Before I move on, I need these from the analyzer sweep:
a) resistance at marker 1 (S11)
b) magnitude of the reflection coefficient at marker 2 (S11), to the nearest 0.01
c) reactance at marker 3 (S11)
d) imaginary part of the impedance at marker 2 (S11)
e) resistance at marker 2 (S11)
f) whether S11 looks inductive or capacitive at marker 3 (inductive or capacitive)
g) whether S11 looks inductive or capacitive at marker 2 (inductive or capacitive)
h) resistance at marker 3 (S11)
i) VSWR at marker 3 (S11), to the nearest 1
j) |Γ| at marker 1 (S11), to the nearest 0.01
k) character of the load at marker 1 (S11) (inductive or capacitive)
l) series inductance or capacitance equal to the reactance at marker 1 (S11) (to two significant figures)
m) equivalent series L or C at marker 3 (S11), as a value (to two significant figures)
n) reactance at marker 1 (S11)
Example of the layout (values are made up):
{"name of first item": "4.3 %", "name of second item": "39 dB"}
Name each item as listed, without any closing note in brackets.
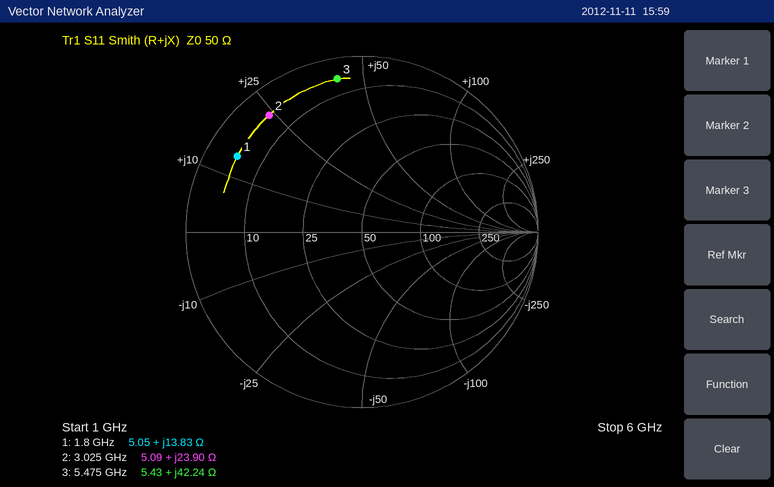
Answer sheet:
{"resistance at marker 1": "5.05 Ω", "magnitude of the reflection coefficient at marker 2 (S11), to the nearest 0.01": "0.85", "reactance at marker 3": "+42.24 Ω", "imaginary part of the impedance at marker 2": "+23.90 Ω", "resistance at marker 2": "5.09 Ω", "whether S11 looks inductive or capacitive at marker 3": "inductive", "whether S11 looks inductive or capacitive at marker 2": "inductive", "resistance at marker 3": "5.43 Ω", "VSWR at marker 3 (S11), to the nearest 1": "16", "|Γ| at marker 1 (S11), to the nearest 0.01": "0.83", "character of the load at marker 1 (S11)": "inductive", "series inductance or capacitance equal to the reactance at marker 1 (S11)": "1.2 nH", "equivalent series L or C at marker 3 (S11), as a value": "1.2 nH", "reactance at marker 1": "+13.83 Ω"}
